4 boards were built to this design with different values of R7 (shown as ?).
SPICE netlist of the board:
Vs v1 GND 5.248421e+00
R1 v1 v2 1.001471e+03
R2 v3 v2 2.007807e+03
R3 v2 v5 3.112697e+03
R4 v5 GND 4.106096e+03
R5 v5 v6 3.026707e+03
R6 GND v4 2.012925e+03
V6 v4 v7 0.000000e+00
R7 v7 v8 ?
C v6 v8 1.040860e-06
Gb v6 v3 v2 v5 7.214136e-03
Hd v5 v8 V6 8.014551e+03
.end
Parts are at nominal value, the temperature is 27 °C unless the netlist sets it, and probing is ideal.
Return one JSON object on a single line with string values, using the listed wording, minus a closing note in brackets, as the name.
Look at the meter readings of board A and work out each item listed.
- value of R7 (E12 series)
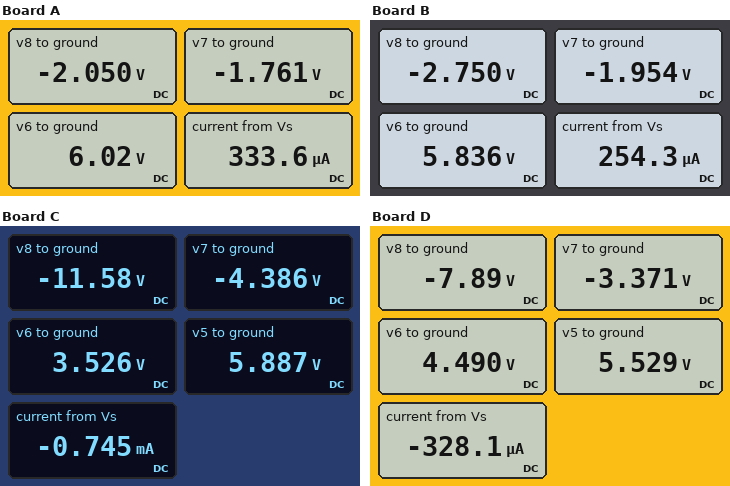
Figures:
{"value of R7": "330 Ω"}
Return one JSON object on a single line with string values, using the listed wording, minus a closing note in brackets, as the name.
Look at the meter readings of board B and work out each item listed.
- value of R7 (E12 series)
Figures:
{"value of R7": "820 Ω"}
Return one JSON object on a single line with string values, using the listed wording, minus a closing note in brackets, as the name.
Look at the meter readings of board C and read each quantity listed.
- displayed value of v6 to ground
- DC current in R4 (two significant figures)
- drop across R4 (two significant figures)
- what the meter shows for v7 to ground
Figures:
{"displayed value of v6 to ground": "3.526 V", "DC current in R4": "1.4 mA", "drop across R4": "5.9 V", "what the meter shows for v7 to ground": "-4.386 V"}
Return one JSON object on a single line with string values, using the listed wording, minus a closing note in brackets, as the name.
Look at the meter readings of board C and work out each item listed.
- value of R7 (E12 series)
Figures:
{"value of R7": "3.3 kΩ"}
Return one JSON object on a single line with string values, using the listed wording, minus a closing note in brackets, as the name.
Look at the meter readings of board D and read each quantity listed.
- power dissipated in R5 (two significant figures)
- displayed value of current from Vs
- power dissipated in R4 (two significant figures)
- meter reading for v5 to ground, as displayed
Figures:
{"power dissipated in R5": "360 µW", "displayed value of current from Vs": "-328.1 µA", "power dissipated in R4": "7.4 mW", "meter reading for v5 to ground, as displayed": "5.529 V"}
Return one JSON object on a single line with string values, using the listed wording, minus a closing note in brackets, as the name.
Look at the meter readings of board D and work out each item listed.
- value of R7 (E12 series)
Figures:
{"value of R7": "2.7 kΩ"}
